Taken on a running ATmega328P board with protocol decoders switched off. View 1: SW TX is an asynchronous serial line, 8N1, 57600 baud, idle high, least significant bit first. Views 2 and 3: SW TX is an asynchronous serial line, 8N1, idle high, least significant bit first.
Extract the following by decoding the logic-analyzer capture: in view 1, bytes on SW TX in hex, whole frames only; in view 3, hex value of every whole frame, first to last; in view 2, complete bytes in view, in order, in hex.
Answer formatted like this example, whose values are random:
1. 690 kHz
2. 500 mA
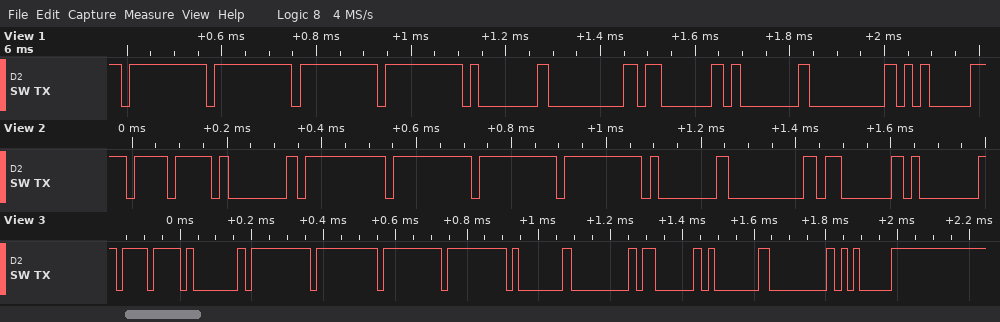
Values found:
1. 0xFF 0xFF 0xFF 0xFF 0x01 0x00 0x03 0x01 0x00 0x05
2. EF 01 FF FF FF FF 01 00 03 01 00 05
3. EF 01 FF FF FF FF 01 00 03 01
